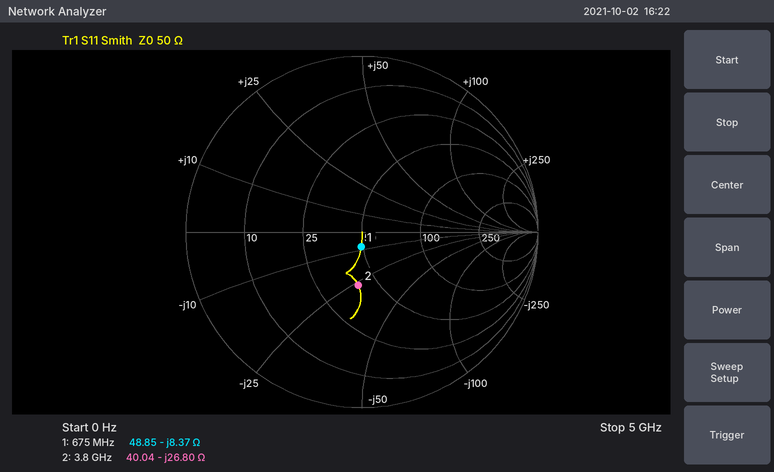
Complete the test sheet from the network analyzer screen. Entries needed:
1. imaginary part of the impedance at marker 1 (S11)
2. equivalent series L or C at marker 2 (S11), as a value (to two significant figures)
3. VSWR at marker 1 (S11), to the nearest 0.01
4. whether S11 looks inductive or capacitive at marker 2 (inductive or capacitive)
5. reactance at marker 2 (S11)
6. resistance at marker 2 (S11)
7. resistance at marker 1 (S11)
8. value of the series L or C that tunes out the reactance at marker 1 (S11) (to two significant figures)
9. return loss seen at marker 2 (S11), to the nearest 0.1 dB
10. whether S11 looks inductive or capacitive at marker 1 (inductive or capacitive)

-8.37 Ω
1.6 pF
1.19
capacitive
-26.80 Ω
40.04 Ω
48.85 Ω
2.0 nH
10.3 dB
capacitive
